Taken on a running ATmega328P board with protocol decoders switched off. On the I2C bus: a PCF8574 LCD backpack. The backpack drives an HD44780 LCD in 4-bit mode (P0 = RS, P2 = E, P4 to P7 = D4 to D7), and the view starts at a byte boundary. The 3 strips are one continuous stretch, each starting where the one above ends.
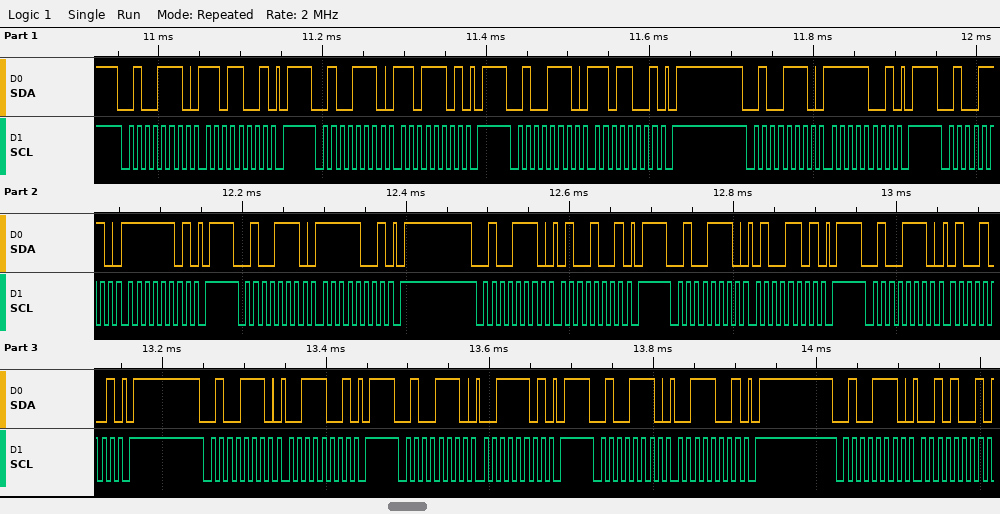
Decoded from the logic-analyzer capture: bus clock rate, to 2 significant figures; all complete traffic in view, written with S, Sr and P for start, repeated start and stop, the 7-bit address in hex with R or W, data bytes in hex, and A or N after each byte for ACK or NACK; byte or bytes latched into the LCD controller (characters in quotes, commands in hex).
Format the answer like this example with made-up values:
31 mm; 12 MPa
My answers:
100 kHz; S 27W A D9 A P S 27W A DD A P S 27W A D9 A P S 27W A F9 A P S 27W A FD A P S 27W A F9 A P S 27W A 49 A P S 27W A 4D A P S 27W A 49 A P S 27W A 39 A P S 27W A 3D A P S 27W A 39 A P S 27W A 29 A; data 0xDF 'C'
